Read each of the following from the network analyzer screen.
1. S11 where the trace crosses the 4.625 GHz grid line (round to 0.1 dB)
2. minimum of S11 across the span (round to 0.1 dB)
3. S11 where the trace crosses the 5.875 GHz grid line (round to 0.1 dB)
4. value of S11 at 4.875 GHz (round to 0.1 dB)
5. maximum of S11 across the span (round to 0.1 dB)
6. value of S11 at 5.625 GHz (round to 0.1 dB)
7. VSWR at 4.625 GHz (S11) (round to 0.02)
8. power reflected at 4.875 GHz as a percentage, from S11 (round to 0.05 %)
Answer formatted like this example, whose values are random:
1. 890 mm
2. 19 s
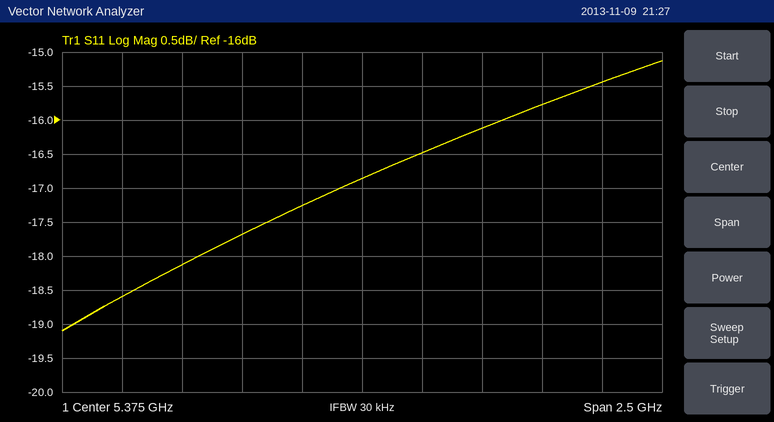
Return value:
1. -18.1 dB
2. -19.1 dB
3. -16.1 dB
4. -17.7 dB
5. -15.1 dB
6. -16.5 dB
7. 1.28
8. 1.70 %
